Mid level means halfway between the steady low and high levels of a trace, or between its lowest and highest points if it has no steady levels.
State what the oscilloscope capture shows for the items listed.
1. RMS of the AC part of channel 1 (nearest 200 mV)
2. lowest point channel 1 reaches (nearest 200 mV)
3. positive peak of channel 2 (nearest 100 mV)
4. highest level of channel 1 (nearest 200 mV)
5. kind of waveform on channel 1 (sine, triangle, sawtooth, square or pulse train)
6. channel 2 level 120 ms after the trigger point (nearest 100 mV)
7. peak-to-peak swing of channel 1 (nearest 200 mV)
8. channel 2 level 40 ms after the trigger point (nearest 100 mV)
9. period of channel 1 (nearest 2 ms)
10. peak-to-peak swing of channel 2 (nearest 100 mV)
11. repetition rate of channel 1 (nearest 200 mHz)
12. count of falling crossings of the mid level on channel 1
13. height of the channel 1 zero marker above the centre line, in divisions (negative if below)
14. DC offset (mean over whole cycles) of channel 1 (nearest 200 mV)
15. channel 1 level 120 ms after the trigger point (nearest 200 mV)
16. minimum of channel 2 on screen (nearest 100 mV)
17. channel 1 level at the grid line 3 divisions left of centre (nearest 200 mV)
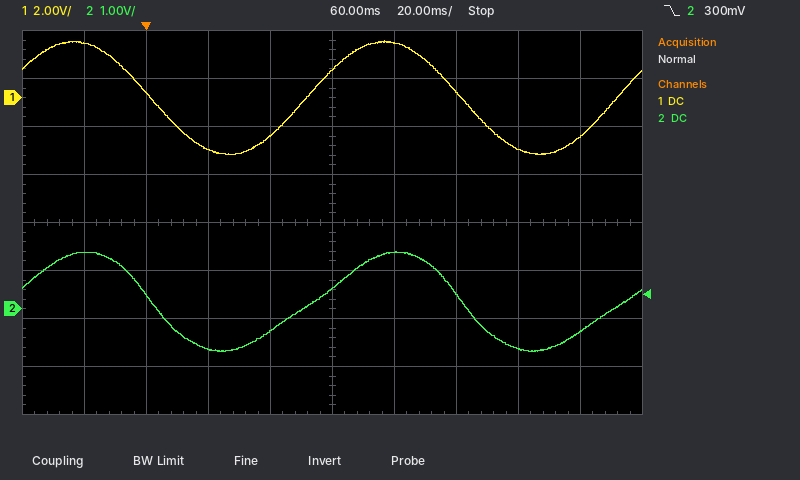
1.6 V
-2.4 V
1.2 V
2.4 V
sine
-800 mV
4.8 V
-500 mV
100 ms
2.1 V
10.0 Hz
2
+2.6 div
0.0 V
-2.2 V
-900 mV
200 mV
